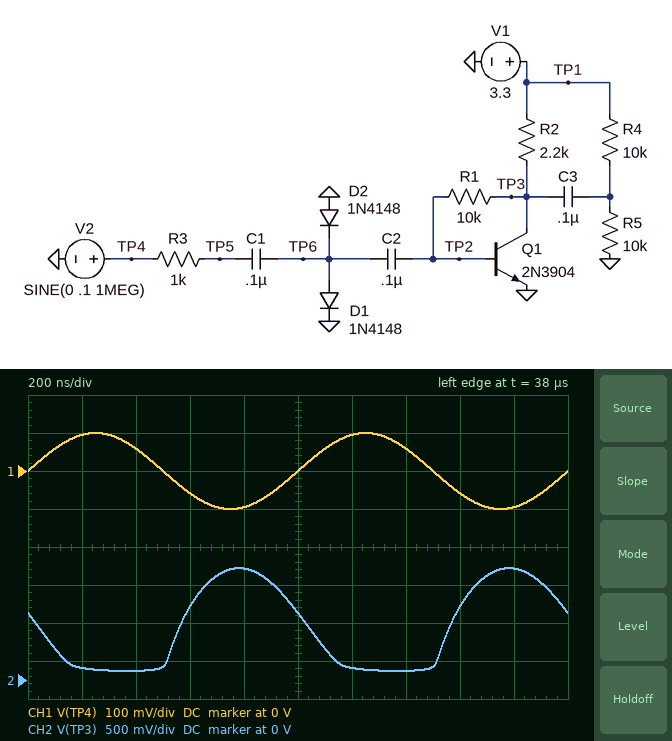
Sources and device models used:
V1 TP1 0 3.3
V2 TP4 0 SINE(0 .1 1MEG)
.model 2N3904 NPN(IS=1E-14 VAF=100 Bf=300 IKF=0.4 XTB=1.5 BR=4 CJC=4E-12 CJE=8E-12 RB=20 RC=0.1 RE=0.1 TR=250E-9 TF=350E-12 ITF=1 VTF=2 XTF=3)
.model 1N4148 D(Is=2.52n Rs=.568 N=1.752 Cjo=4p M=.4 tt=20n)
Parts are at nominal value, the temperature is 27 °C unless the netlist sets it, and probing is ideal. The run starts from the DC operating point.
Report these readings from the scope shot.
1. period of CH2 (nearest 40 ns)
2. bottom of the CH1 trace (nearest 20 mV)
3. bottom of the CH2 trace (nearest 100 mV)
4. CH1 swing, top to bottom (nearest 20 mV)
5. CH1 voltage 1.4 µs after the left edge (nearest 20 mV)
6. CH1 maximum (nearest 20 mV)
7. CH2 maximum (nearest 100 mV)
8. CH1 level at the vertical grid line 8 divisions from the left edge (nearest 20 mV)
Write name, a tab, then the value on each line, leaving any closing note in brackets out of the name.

period of CH2	1.00 µs
bottom of the CH1 trace	-100 mV
bottom of the CH2 trace	100 mV
CH1 swing, top to bottom	200 mV
CH1 voltage 1.4 µs after the left edge	60 mV
CH1 maximum	100 mV
CH2 maximum	1.5 V
CH1 level at the vertical grid line 8 divisions from the left edge	-60 mV
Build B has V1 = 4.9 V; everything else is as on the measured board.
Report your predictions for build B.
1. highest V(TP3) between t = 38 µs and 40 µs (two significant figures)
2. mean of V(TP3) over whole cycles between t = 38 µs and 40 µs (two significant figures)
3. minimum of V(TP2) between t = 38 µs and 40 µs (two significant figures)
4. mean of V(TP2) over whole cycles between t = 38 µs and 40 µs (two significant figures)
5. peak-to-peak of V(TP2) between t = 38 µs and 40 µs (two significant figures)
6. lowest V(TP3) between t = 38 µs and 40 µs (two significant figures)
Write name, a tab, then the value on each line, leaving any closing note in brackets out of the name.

highest V(TP3) between t = 38 µs and 40 µs	1.6 V
mean of V(TP3) over whole cycles between t = 38 µs and 40 µs	740 mV
minimum of V(TP2) between t = 38 µs and 40 µs	660 mV
mean of V(TP2) over whole cycles between t = 38 µs and 40 µs	670 mV
peak-to-peak of V(TP2) between t = 38 µs and 40 µs	18 mV
lowest V(TP3) between t = 38 µs and 40 µs	130 mV
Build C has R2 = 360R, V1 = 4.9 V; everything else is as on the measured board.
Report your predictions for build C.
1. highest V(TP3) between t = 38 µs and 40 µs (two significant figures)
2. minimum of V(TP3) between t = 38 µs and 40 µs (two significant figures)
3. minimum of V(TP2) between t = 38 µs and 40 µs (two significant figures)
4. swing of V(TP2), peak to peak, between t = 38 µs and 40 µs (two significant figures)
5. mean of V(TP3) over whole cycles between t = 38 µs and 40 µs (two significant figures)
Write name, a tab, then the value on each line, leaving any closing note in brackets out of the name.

highest V(TP3) between t = 38 µs and 40 µs	1.9 V
minimum of V(TP3) between t = 38 µs and 40 µs	290 mV
minimum of V(TP2) between t = 38 µs and 40 µs	710 mV
swing of V(TP2), peak to peak, between t = 38 µs and 40 µs	14 mV
mean of V(TP3) over whole cycles between t = 38 µs and 40 µs	1.1 V
